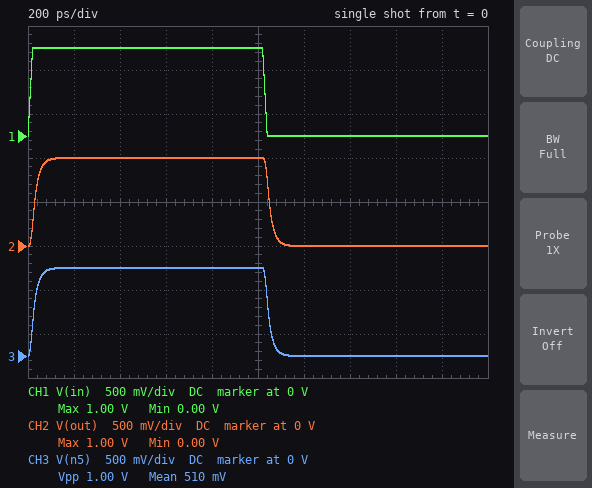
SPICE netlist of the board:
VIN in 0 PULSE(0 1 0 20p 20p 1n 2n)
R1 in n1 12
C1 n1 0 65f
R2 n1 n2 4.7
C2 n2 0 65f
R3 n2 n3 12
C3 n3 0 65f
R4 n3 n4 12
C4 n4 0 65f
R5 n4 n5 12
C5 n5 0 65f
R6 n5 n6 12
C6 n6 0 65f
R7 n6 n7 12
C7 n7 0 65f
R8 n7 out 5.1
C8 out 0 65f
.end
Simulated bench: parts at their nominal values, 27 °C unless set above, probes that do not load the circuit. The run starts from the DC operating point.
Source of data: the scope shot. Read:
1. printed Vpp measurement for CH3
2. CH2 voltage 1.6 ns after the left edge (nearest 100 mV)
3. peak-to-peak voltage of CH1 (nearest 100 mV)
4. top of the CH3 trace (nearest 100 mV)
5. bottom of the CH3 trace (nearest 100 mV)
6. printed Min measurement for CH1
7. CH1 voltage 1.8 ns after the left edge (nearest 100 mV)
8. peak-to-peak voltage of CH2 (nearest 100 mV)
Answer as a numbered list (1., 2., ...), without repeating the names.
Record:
1. 1.00 V
2. 0 V
3. 1.0 V
4. 1.0 V
5. 0 V
6. 0.00 V
7. 0 V
8. 1.0 V
